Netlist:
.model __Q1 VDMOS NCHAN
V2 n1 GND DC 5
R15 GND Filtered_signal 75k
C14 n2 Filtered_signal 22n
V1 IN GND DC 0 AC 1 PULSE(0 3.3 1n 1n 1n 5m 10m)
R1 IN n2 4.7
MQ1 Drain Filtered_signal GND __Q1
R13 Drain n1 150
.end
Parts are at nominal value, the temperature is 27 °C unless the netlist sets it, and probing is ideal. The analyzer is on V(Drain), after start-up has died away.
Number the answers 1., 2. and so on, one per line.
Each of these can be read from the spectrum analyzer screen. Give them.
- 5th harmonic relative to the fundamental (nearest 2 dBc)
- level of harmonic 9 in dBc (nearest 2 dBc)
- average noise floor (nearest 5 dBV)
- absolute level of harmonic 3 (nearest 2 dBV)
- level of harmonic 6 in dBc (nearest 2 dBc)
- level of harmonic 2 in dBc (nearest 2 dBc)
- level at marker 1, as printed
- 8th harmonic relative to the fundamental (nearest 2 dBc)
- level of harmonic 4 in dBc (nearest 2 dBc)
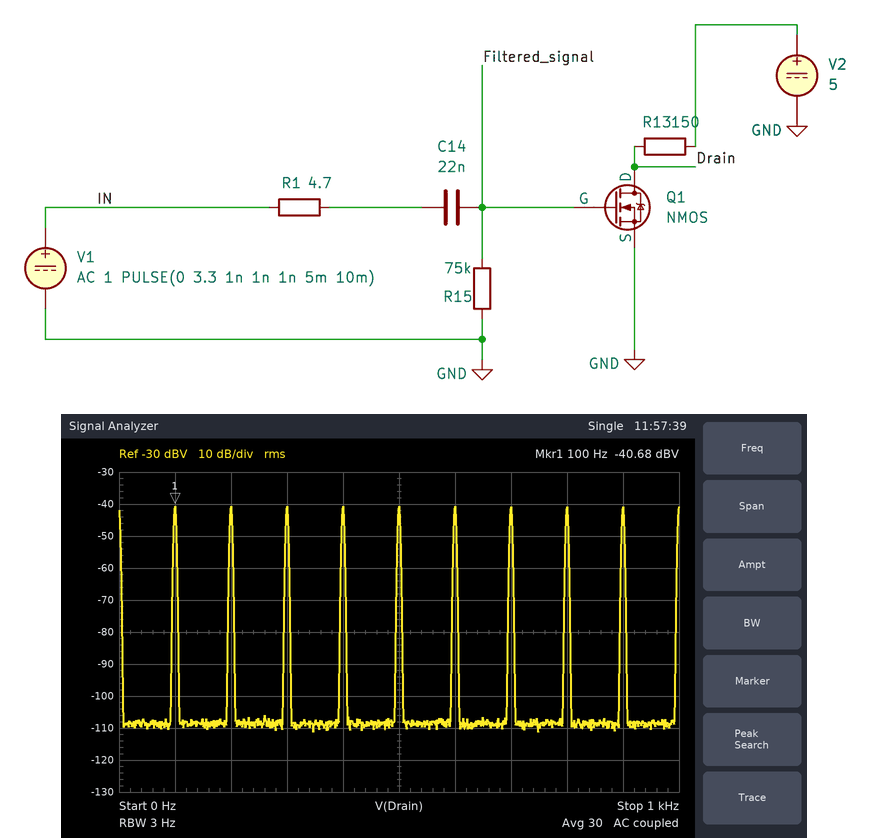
1. 0 dBc
2. 0 dBc
3. -110 dBV
4. -40 dBV
5. 0 dBc
6. 0 dBc
7. -40.68 dBV
8. 0 dBc
9. 0 dBc
